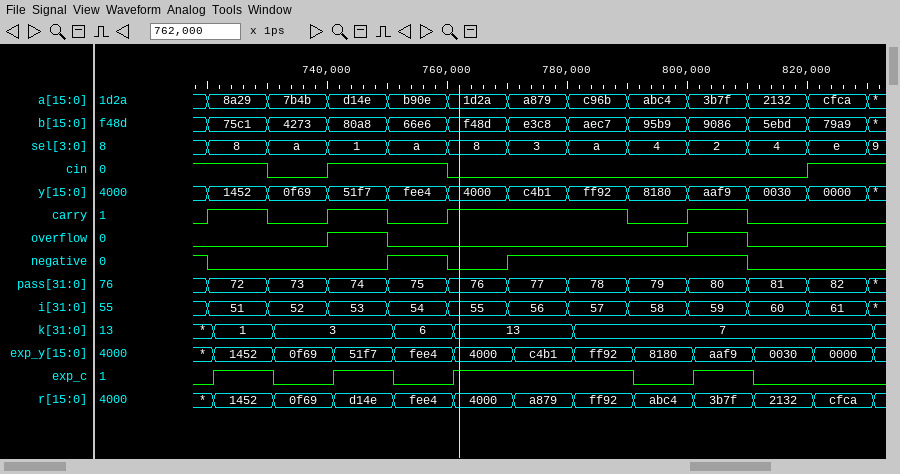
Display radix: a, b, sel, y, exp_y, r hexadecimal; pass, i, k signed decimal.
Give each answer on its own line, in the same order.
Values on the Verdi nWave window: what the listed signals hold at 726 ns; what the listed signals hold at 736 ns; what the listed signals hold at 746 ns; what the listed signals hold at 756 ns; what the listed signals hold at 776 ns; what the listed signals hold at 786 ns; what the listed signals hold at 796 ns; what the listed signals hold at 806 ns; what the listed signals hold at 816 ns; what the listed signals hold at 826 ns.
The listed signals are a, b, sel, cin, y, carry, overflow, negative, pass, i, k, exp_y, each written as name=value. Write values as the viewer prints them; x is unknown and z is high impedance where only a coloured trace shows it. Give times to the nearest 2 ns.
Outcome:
a=8a29, b=75c1, sel=8, cin=1, y=1452, carry=1, overflow=0, negative=0, pass=72, i=51, k=1, exp_y=1452
a=7b4b, b=4273, sel=a, cin=0, y=0f69, carry=0, overflow=0, negative=0, pass=73, i=52, k=3, exp_y=0f69
a=d14e, b=80a8, sel=1, cin=1, y=51f7, carry=1, overflow=1, negative=0, pass=74, i=53, k=3, exp_y=51f7
a=b90e, b=66e6, sel=a, cin=1, y=fee4, carry=0, overflow=0, negative=1, pass=75, i=54, k=6, exp_y=fee4
a=a879, b=e3c8, sel=3, cin=0, y=c4b1, carry=1, overflow=0, negative=1, pass=77, i=56, k=13, exp_y=c4b1
a=c96b, b=aec7, sel=a, cin=0, y=ff92, carry=1, overflow=0, negative=1, pass=78, i=57, k=7, exp_y=ff92
a=abc4, b=95b9, sel=4, cin=0, y=8180, carry=0, overflow=0, negative=1, pass=79, i=58, k=7, exp_y=8180
a=3b7f, b=9086, sel=2, cin=0, y=aaf9, carry=1, overflow=1, negative=1, pass=80, i=59, k=7, exp_y=aaf9
a=2132, b=5ebd, sel=4, cin=0, y=0030, carry=0, overflow=0, negative=0, pass=81, i=60, k=7, exp_y=0030
a=cfca, b=79a9, sel=e, cin=1, y=0000, carry=0, overflow=0, negative=0, pass=82, i=61, k=7, exp_y=0000
